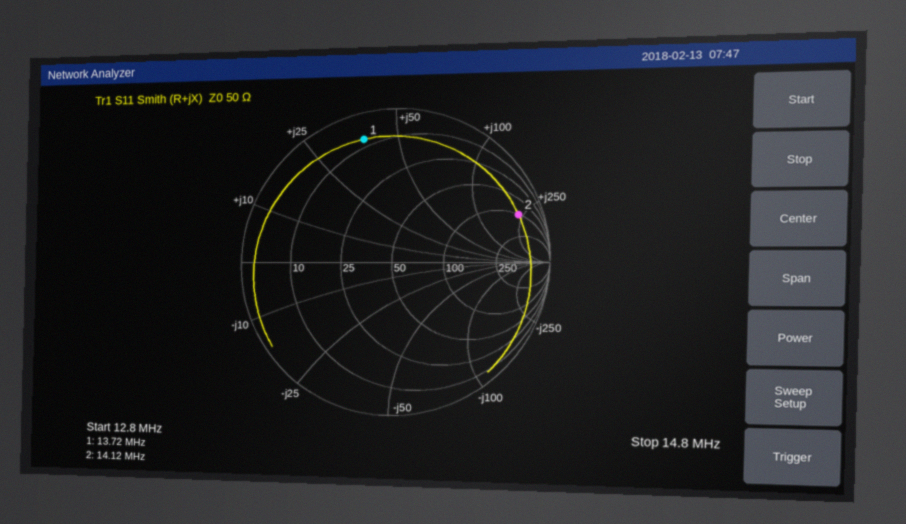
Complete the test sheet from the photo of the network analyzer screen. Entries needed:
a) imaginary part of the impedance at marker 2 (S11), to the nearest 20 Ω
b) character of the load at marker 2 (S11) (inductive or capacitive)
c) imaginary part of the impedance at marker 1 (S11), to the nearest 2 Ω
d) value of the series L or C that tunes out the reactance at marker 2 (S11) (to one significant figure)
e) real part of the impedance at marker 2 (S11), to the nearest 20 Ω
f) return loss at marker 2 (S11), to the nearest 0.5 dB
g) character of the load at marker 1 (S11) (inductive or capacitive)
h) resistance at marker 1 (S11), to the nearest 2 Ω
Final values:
+220 Ω
inductive
+38 Ω
50 pF
100 Ω
1.5 dB
inductive
8 Ω
